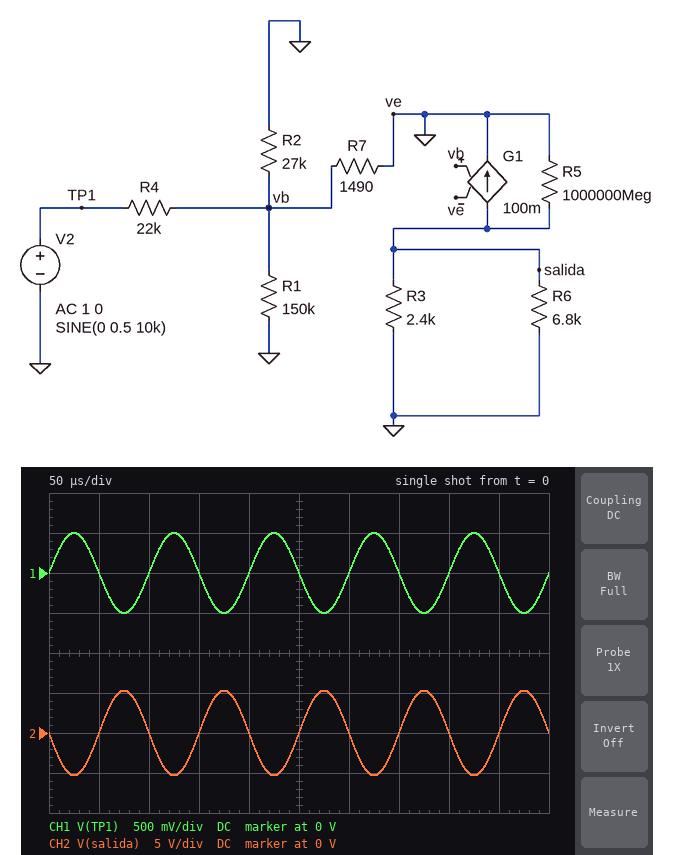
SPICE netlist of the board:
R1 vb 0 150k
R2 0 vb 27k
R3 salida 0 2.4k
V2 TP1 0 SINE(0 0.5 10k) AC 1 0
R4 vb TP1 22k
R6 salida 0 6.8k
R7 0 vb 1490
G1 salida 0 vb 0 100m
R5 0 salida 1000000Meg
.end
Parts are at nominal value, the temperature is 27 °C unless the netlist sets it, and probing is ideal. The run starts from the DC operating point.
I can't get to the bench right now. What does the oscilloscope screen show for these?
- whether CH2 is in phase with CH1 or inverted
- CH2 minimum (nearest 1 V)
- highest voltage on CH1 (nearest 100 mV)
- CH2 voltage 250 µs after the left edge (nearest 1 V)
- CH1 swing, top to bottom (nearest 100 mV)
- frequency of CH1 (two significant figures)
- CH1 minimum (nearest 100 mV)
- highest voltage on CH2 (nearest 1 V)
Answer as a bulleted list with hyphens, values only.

- inverted
- -5 V
- 500 mV
- 0 V
- 1.0 V
- 10 kHz
- -500 mV
- 5 V
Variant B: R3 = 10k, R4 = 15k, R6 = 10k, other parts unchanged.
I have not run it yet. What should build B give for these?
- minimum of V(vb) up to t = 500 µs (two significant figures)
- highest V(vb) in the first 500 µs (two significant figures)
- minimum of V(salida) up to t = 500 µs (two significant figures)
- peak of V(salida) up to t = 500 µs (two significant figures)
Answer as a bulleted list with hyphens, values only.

- -43 mV
- 43 mV
- -21 V
- 21 V
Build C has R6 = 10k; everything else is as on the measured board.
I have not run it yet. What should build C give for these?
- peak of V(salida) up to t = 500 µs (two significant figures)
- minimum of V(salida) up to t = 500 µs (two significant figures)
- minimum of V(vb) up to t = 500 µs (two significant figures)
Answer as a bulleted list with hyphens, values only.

- 5.8 V
- -5.8 V
- -30 mV
